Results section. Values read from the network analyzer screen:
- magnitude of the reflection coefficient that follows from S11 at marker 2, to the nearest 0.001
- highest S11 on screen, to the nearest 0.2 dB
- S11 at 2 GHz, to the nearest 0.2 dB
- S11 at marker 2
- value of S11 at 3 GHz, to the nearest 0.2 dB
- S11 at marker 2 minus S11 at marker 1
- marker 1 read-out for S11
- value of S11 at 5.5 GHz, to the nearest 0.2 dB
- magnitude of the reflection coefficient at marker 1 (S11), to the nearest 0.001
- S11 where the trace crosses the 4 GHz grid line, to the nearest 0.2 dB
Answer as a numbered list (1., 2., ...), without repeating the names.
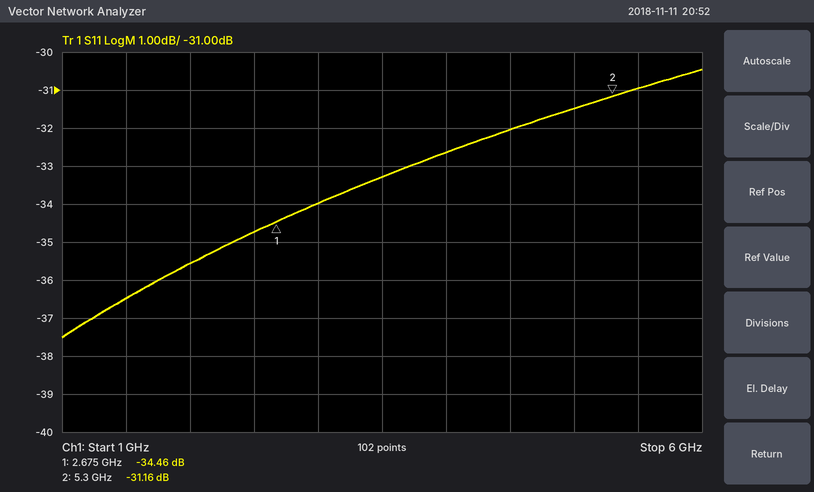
1. 0.028
2. -30.4 dB
3. -35.6 dB
4. -31.16 dB
5. -34.0 dB
6. 3.30 dB
7. -34.46 dB
8. -31.0 dB
9. 0.019
10. -32.6 dB
